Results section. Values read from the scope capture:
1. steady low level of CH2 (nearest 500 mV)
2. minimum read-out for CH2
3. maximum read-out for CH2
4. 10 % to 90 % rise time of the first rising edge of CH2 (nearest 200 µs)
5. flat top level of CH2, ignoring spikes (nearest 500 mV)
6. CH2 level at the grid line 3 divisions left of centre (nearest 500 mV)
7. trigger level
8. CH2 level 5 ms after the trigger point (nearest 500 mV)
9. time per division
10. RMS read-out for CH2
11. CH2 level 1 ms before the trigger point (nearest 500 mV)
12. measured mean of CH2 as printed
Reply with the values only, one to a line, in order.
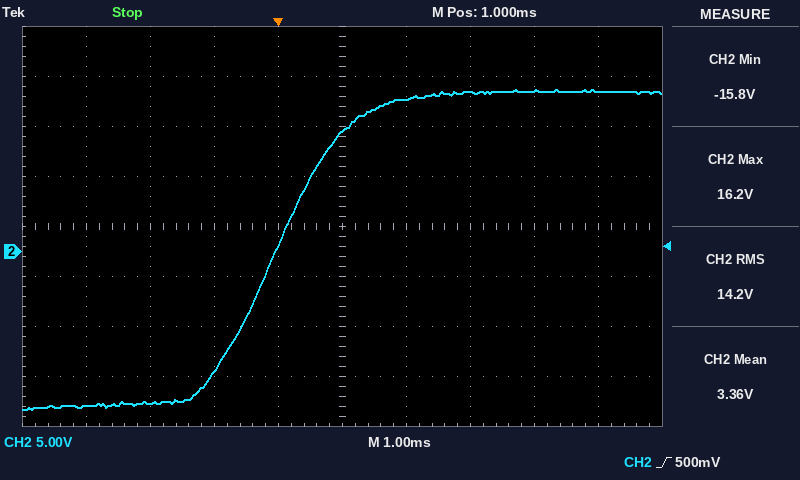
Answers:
-15.5 V
-15.8 V
16.2 V
2.2 ms
16.0 V
-15.0 V
500 mV
16.0 V
1 ms
14.2 V
-12.0 V
3.36 V
